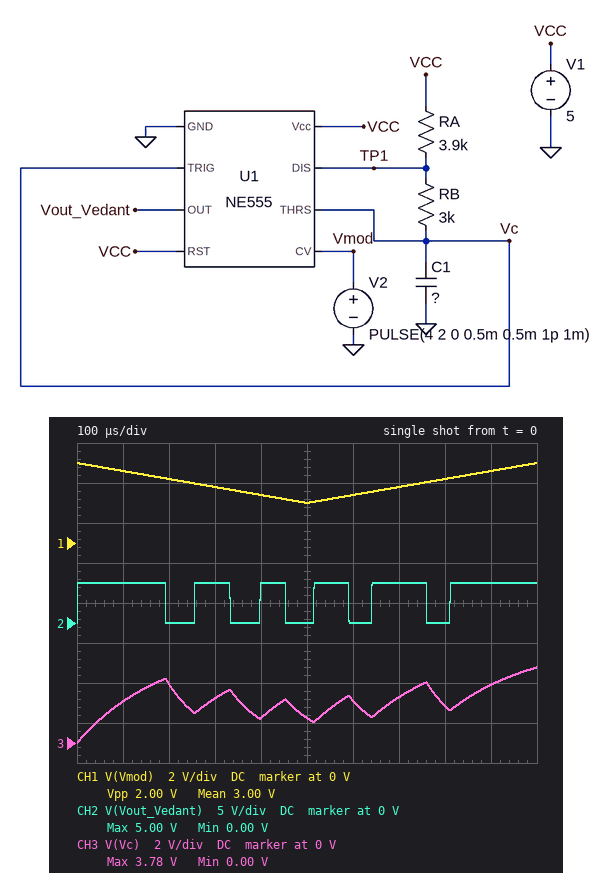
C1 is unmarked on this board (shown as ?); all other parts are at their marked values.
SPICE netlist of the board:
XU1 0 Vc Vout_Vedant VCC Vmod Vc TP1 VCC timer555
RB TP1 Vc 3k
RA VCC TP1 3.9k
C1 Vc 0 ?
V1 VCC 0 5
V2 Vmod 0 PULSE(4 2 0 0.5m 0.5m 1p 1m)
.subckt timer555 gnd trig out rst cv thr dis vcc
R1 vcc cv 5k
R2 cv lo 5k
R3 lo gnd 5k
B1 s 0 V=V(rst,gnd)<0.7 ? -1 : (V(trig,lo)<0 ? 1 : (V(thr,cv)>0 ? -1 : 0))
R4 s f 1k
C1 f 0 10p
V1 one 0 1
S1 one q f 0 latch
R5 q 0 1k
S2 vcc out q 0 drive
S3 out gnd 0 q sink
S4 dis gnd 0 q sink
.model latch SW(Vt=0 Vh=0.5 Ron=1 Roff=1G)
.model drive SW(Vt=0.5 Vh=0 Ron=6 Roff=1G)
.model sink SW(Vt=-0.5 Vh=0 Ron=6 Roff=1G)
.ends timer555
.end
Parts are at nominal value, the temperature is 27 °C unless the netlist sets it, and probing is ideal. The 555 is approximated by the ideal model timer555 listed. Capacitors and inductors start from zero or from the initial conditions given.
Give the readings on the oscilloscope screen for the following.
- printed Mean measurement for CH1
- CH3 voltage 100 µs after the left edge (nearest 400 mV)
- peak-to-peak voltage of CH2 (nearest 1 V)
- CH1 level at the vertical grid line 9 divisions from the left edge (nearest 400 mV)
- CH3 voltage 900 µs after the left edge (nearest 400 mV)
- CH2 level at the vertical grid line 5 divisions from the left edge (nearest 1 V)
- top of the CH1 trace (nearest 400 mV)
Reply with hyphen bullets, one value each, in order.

- 3.00 V
- 2.0 V
- 5 V
- 3.6 V
- 2.8 V
- 0 V
- 4.0 V
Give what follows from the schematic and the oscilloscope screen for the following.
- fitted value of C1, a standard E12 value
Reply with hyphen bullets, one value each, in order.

- 27 nF
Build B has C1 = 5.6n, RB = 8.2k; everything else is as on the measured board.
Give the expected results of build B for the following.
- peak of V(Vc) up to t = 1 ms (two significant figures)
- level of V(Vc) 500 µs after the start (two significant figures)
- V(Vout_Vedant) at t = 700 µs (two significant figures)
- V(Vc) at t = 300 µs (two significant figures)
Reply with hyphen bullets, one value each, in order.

- 3.9 V
- 1.3 V
- 5.0 V
- 2.6 V
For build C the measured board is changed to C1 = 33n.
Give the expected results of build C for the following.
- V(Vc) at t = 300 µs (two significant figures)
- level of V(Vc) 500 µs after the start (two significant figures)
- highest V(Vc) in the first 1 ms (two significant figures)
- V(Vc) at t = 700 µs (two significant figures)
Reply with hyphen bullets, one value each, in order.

- 1.4 V
- 1.6 V
- 3.6 V
- 2.6 V
